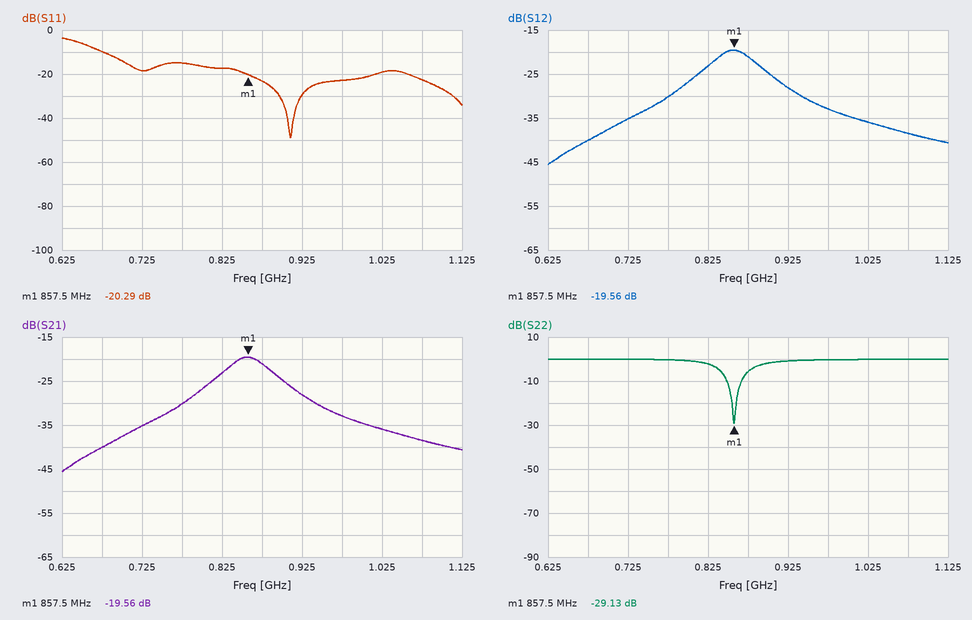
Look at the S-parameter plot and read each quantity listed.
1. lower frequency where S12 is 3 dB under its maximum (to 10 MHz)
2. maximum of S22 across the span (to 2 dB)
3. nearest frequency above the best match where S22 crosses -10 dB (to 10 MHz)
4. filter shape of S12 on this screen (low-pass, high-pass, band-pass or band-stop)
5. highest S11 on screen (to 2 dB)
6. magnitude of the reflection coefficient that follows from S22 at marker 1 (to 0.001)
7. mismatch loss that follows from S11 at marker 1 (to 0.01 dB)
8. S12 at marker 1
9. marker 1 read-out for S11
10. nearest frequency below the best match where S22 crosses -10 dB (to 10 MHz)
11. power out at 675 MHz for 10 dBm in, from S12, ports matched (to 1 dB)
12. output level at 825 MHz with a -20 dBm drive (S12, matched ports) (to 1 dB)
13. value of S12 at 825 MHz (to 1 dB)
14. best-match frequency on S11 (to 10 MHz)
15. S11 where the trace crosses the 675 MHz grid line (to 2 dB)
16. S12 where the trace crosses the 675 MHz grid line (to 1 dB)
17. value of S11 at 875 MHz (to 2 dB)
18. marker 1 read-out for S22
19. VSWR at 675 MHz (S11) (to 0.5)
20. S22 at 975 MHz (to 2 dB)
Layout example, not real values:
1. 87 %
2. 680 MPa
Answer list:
1. 830 MHz
2. 0 dB
3. 870 MHz
4. band-pass
5. -4 dB
6. 0.035
7. 0.04 dB
8. -19.56 dB
9. -20.29 dB
10. 850 MHz
11. -30 dBm
12. -43 dBm
13. -23 dB
14. 910 MHz
15. -10 dB
16. -40 dB
17. -24 dB
18. -29.13 dB
19. 2.0
20. 0 dB
